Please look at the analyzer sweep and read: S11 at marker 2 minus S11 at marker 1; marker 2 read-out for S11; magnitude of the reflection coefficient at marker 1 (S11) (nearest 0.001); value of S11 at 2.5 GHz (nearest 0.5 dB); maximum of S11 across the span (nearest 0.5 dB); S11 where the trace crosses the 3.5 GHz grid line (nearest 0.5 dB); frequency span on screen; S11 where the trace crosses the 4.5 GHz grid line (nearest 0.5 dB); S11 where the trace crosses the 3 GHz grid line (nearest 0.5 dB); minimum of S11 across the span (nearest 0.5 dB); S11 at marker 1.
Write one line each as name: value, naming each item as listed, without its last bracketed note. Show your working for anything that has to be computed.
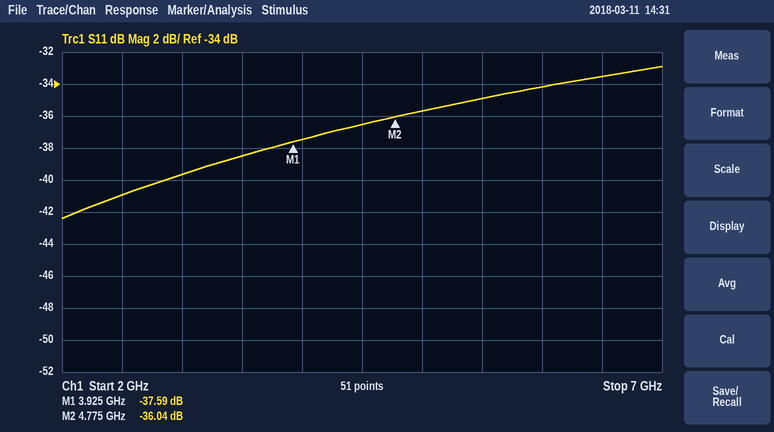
S11 at marker 2 minus S11 at marker 1: -36.04 − (-37.59) = 1.55 dB
marker 2 read-out for S11: -36.04 dB
magnitude of the reflection coefficient at marker 1 (S11): 10^(-37.59/20) ≈ 0.013
value of S11 at 2.5 GHz: -41.0 dB
maximum of S11 across the span: -33.0 dB
S11 where the trace crosses the 3.5 GHz grid line: -38.5 dB
frequency span on screen: 5 GHz
S11 where the trace crosses the 4.5 GHz grid line: -36.5 dB
S11 where the trace crosses the 3 GHz grid line: -39.5 dB
minimum of S11 across the span: -42.5 dB
S11 at marker 1: -37.59 dB
